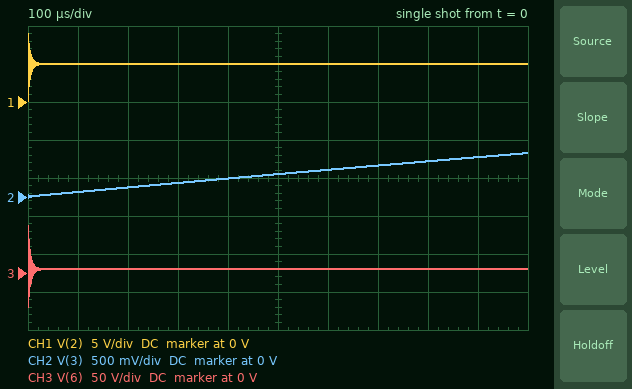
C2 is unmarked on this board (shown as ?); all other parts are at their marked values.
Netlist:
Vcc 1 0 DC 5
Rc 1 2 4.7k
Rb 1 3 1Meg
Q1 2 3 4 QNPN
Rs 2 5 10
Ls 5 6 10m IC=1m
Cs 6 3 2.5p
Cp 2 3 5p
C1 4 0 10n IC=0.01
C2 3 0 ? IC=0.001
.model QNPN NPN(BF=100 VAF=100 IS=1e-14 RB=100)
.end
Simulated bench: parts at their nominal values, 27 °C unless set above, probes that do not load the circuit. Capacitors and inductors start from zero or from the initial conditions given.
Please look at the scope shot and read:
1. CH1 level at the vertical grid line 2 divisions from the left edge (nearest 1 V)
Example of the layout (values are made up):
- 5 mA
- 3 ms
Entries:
- 5 V
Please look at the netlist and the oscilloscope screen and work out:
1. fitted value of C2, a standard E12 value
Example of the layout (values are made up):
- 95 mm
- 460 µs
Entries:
- 8.2 nF
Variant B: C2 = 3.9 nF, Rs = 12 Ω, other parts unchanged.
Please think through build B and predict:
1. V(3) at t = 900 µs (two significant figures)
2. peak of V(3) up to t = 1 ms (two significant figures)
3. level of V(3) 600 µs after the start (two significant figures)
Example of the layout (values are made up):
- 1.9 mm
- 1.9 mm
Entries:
- 1.0 V
- 1.1 V
- 720 mV
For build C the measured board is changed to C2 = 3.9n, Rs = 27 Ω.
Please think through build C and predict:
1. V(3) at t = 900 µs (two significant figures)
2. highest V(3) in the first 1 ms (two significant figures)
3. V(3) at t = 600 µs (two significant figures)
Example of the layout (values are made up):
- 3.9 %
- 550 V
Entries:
- 1.0 V
- 1.1 V
- 720 mV
